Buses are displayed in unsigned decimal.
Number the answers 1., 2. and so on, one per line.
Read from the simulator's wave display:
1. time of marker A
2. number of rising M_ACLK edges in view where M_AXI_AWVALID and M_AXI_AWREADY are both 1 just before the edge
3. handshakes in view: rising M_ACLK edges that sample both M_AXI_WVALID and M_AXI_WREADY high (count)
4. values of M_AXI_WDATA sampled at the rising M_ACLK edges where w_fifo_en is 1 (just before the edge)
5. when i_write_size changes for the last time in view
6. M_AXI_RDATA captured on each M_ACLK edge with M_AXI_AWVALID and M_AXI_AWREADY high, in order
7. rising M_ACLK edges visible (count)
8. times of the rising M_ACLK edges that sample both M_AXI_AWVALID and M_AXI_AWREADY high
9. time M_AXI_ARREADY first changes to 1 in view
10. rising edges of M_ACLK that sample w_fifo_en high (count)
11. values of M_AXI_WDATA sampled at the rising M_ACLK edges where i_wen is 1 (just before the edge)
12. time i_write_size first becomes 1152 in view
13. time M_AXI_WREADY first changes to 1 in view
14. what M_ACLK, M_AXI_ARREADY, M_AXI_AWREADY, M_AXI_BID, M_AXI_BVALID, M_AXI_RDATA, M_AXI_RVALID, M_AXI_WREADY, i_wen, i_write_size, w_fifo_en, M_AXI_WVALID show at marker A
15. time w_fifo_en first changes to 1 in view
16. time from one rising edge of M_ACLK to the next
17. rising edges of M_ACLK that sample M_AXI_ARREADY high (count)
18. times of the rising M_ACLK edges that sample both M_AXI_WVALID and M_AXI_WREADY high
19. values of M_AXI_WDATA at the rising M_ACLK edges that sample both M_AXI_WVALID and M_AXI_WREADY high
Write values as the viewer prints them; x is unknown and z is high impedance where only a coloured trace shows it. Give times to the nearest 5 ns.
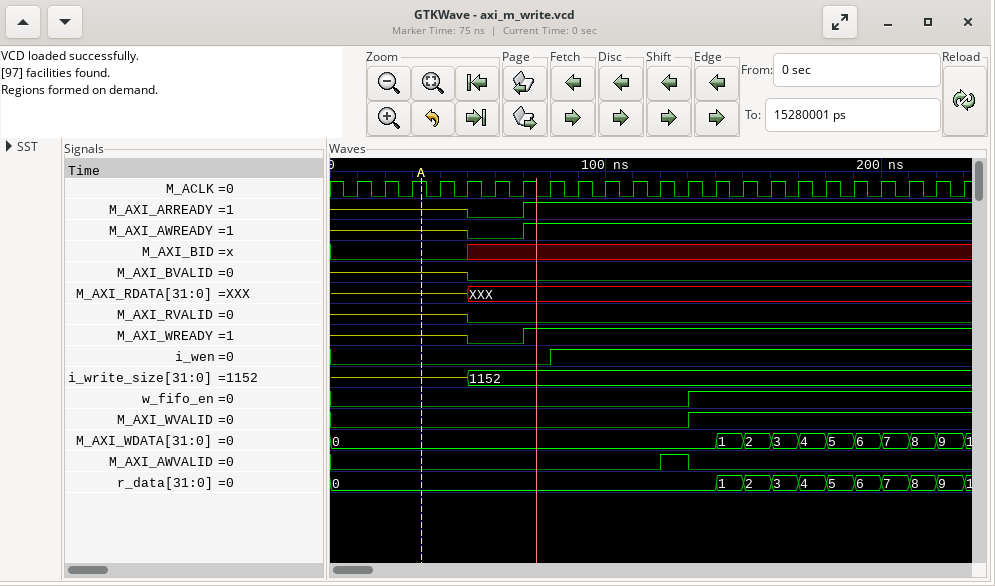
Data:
1. 35 ns
2. 1
3. 10
4. 0, 1, 2, 3, 4, 5, 6, 7, 8, 9
5. 50 ns
6. XXX
7. 23
8. 130 ns
9. 70 ns
10. 10
11. 0, 0, 0, 0, 0, 0, 1, 2, 3, 4, 5, 6, 7, 8, 9
12. 50 ns
13. 70 ns
14. M_ACLK=1, M_AXI_ARREADY=z, M_AXI_AWREADY=z, M_AXI_BID=0, M_AXI_BVALID=z, M_AXI_RDATA=z, M_AXI_RVALID=z, M_AXI_WREADY=z, i_wen=0, i_write_size=z, w_fifo_en=0, M_AXI_WVALID=0
15. 130 ns
16. 10 ns
17. 16
18. 140 ns, 150 ns, 160 ns, 170 ns, 180 ns, 190 ns, 200 ns, 210 ns, 220 ns, 230 ns
19. 0, 1, 2, 3, 4, 5, 6, 7, 8, 9
